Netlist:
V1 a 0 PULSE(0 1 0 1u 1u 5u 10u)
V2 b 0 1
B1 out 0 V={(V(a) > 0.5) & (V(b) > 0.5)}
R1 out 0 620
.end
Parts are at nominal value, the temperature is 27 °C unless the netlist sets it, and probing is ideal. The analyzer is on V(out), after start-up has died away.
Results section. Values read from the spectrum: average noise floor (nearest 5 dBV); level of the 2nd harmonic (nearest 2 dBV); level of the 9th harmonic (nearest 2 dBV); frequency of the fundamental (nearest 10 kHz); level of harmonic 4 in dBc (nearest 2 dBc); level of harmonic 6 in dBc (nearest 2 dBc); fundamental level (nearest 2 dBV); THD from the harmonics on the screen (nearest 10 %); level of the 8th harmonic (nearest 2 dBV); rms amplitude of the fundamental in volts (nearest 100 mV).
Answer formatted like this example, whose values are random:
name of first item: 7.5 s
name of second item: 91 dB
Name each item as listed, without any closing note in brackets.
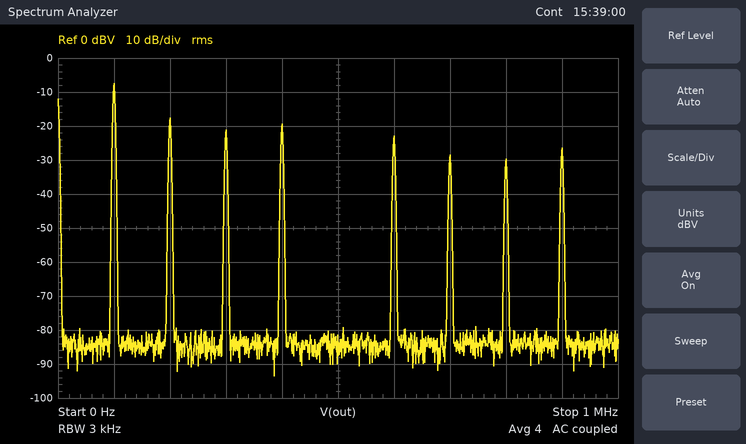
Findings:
average noise floor: -85 dBV
level of the 2nd harmonic: -18 dBV
level of the 9th harmonic: -26 dBV
frequency of the fundamental: 100 kHz
level of harmonic 4 in dBc: -12 dBc
level of harmonic 6 in dBc: -16 dBc
fundamental level: -8 dBV
THD from the harmonics on the screen: 50 %
level of the 8th harmonic: -30 dBV
rms amplitude of the fundamental in volts: 400 mV
